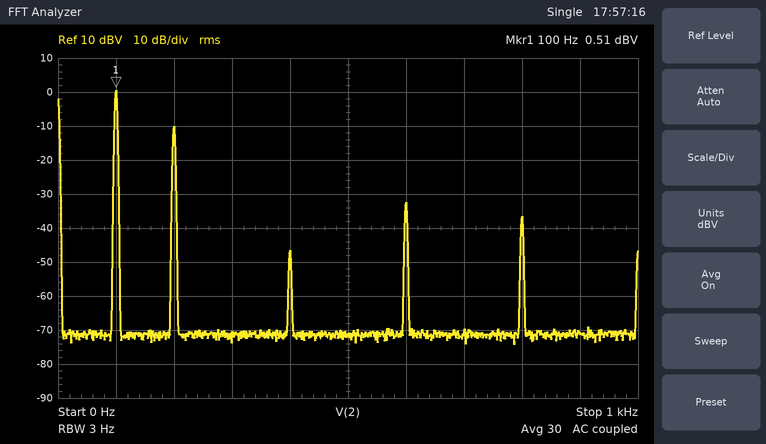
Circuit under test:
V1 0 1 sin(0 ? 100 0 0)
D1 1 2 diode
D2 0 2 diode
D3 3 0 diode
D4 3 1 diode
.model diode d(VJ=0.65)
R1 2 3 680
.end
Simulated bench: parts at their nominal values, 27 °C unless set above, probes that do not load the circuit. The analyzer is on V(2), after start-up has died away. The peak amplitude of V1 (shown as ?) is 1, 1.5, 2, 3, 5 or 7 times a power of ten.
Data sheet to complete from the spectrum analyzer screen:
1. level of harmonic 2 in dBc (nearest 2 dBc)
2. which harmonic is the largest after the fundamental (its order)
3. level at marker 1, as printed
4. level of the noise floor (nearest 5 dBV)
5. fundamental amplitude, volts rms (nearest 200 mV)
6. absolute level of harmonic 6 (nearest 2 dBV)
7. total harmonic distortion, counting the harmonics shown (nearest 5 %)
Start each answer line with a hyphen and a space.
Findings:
- -10 dBc
- 2
- 0.51 dBV
- -70 dBV
- 1.0 V
- -32 dBV
- 30 %
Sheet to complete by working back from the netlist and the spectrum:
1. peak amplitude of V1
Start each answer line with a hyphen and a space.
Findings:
- 3 V
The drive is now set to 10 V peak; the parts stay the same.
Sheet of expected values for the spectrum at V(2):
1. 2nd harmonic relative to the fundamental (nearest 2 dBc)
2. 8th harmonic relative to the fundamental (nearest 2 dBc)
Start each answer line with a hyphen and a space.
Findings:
- -8 dBc
- -40 dBc
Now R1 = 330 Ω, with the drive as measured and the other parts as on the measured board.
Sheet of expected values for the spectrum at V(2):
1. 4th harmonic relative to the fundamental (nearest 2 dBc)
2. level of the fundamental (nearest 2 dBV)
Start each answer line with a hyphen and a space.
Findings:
- -42 dBc
- 0 dBV
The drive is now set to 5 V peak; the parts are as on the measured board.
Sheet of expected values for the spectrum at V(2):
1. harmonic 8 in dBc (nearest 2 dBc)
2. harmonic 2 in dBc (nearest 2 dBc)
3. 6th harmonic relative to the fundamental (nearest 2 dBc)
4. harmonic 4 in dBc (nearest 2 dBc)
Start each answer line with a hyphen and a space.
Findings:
- -42 dBc
- -8 dBc
- -56 dBc
- -28 dBc
